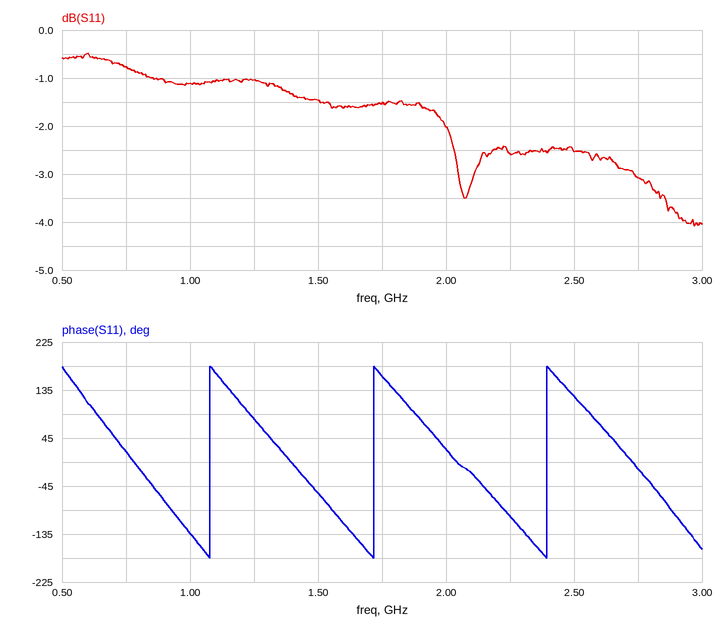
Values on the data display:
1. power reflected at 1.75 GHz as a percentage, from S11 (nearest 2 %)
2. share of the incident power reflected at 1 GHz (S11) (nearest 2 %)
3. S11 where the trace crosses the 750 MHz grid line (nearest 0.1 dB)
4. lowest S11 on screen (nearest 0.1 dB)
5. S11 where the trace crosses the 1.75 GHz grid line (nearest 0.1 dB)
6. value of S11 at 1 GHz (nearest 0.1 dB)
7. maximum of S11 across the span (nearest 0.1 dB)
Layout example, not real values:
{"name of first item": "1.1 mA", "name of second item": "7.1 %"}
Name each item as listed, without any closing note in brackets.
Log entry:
{"power reflected at 1.75 GHz as a percentage, from S11": "70 %", "share of the incident power reflected at 1 GHz (S11)": "78 %", "S11 where the trace crosses the 750 MHz grid line": "-0.8 dB", "lowest S11 on screen": "-4.1 dB", "S11 where the trace crosses the 1.75 GHz grid line": "-1.5 dB", "value of S11 at 1 GHz": "-1.1 dB", "maximum of S11 across the span": "-0.5 dB"}
